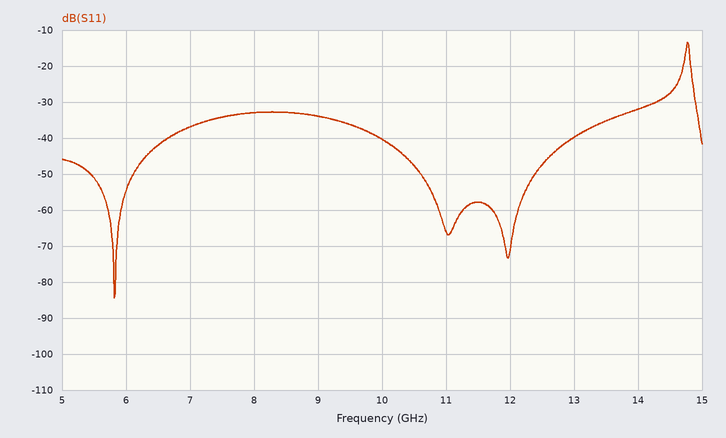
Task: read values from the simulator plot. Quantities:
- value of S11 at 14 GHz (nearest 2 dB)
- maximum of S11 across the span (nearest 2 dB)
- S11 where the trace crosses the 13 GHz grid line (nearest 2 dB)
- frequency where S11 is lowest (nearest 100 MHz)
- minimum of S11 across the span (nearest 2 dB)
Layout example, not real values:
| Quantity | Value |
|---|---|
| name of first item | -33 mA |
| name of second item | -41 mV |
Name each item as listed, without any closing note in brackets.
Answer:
| Quantity | Value |
|---|---|
| value of S11 at 14 GHz | -32 dB |
| maximum of S11 across the span | -14 dB |
| S11 where the trace crosses the 13 GHz grid line | -40 dB |
| frequency where S11 is lowest | 5.8 GHz |
| minimum of S11 across the span | -84 dB |
